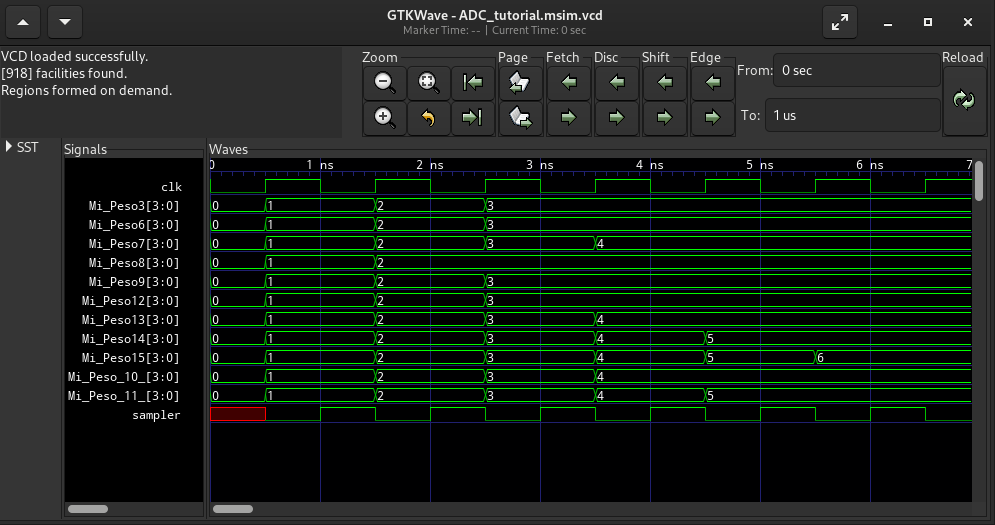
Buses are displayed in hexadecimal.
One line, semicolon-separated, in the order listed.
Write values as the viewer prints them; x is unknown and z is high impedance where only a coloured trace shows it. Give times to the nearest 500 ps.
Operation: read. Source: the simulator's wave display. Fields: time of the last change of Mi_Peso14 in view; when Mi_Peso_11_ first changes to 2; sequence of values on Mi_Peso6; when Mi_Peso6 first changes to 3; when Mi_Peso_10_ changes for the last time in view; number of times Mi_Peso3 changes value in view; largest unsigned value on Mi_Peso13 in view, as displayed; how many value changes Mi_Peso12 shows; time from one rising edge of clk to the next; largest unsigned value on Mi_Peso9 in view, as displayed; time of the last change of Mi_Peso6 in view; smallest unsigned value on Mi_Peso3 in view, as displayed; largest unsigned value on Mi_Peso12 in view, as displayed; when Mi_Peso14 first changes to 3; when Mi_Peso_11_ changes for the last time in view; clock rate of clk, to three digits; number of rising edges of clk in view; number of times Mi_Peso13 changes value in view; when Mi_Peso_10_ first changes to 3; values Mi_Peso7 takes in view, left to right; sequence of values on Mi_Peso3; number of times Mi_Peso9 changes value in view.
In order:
4500 ps; 1500 ps; 0, 1, 2, 3; 2500 ps; 3500 ps; 3; 4; 3; 1000 ps; 3; 2500 ps; 0; 3; 2500 ps; 4500 ps; 1.00 GHz; 7; 4; 2500 ps; 0, 1, 2, 3, 4; 0, 1, 2, 3; 3
